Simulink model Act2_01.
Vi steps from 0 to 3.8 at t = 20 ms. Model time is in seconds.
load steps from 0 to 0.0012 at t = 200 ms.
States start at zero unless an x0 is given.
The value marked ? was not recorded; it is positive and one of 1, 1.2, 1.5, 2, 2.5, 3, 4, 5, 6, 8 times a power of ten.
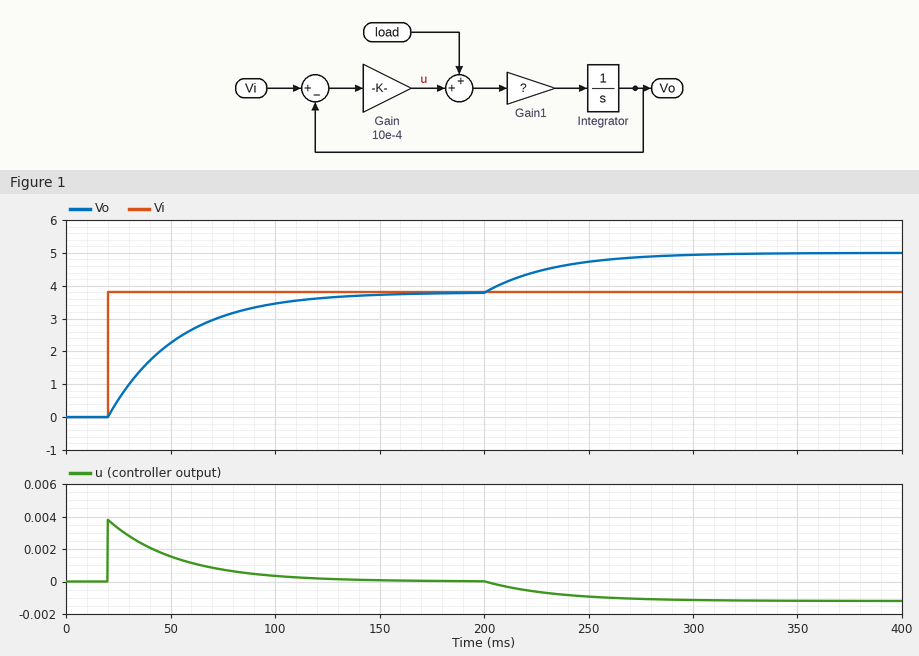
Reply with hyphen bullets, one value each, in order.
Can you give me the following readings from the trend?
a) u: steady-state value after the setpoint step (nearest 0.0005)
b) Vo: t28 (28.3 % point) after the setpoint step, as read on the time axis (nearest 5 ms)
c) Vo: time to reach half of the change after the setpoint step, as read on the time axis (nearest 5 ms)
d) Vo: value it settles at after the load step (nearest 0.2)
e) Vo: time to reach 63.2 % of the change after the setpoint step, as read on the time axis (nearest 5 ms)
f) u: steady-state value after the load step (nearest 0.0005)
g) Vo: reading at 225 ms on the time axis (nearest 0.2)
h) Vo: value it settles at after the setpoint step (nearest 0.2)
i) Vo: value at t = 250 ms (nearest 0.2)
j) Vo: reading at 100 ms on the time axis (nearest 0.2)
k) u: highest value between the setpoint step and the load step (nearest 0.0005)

- 0.0000
- 30 ms
- 45 ms
- 5.0
- 55 ms
- -0.0010
- 4.4
- 3.8
- 4.8
- 3.4
- 0.0040
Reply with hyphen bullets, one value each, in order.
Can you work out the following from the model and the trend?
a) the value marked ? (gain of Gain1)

- 30000
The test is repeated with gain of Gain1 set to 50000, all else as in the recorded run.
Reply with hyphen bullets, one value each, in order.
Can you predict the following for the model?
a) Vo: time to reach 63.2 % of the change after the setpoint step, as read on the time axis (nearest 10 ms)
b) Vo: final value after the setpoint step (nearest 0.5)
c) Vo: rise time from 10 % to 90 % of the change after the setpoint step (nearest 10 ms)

- 40 ms
- 4.0
- 40 ms
